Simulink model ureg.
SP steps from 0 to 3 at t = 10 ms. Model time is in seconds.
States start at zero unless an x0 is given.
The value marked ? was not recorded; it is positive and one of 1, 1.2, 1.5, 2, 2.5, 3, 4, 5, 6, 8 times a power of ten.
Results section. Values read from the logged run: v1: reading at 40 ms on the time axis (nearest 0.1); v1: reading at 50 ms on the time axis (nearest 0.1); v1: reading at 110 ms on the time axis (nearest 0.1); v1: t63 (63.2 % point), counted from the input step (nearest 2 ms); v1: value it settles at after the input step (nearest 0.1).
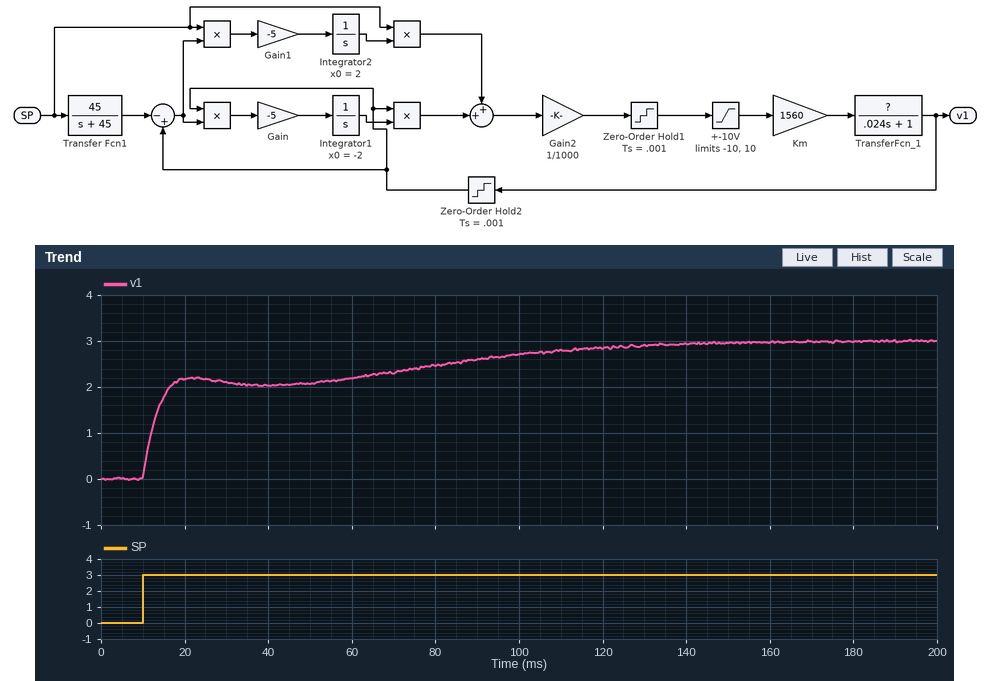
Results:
2.0
2.1
2.8
6 ms
3.0
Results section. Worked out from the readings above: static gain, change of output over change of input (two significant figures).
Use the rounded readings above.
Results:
1.0
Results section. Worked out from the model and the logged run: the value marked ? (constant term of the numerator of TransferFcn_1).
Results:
1.5
